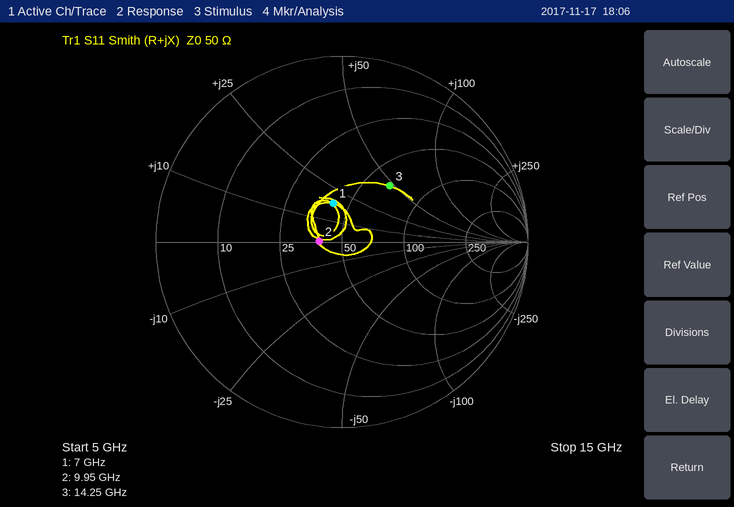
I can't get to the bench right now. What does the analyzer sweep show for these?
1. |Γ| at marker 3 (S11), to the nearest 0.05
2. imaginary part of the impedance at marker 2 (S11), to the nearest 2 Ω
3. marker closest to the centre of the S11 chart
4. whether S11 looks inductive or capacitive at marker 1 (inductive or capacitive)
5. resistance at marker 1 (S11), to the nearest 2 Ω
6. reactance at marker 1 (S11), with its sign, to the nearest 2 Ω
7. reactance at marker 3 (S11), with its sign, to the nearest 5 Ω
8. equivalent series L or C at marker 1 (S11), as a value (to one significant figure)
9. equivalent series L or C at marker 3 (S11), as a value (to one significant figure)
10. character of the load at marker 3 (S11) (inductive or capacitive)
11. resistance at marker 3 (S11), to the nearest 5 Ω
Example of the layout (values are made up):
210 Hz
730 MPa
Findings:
0.40
0 Ω
marker 2
inductive
42 Ω
+18 Ω
+45 Ω
400 pH
500 pH
inductive
65 Ω
